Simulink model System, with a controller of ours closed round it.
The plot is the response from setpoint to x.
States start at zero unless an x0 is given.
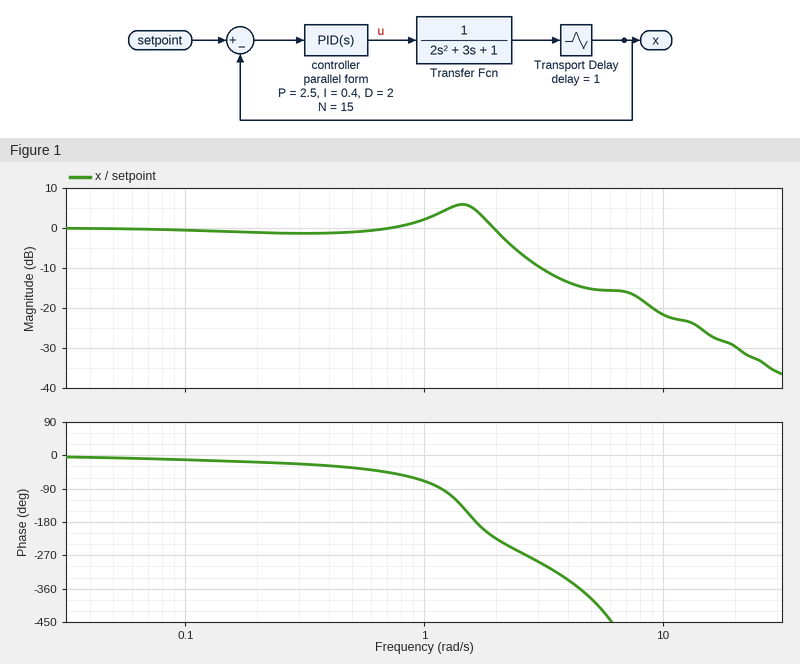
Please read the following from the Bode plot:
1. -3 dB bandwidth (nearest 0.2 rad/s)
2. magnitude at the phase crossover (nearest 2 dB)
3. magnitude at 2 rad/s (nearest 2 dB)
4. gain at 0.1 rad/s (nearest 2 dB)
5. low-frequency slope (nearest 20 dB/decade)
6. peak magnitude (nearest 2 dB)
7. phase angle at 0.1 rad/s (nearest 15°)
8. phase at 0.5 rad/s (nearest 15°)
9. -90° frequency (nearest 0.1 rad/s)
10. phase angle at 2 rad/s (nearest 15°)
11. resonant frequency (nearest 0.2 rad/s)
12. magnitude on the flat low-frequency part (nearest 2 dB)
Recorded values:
2.2 rad/s
4 dB
0 dB
0 dB
0 dB/decade
6 dB
-15°
-30°
1.2 rad/s
-225°
1.4 rad/s
0 dB
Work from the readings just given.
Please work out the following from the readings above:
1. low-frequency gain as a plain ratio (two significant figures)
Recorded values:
1.0
